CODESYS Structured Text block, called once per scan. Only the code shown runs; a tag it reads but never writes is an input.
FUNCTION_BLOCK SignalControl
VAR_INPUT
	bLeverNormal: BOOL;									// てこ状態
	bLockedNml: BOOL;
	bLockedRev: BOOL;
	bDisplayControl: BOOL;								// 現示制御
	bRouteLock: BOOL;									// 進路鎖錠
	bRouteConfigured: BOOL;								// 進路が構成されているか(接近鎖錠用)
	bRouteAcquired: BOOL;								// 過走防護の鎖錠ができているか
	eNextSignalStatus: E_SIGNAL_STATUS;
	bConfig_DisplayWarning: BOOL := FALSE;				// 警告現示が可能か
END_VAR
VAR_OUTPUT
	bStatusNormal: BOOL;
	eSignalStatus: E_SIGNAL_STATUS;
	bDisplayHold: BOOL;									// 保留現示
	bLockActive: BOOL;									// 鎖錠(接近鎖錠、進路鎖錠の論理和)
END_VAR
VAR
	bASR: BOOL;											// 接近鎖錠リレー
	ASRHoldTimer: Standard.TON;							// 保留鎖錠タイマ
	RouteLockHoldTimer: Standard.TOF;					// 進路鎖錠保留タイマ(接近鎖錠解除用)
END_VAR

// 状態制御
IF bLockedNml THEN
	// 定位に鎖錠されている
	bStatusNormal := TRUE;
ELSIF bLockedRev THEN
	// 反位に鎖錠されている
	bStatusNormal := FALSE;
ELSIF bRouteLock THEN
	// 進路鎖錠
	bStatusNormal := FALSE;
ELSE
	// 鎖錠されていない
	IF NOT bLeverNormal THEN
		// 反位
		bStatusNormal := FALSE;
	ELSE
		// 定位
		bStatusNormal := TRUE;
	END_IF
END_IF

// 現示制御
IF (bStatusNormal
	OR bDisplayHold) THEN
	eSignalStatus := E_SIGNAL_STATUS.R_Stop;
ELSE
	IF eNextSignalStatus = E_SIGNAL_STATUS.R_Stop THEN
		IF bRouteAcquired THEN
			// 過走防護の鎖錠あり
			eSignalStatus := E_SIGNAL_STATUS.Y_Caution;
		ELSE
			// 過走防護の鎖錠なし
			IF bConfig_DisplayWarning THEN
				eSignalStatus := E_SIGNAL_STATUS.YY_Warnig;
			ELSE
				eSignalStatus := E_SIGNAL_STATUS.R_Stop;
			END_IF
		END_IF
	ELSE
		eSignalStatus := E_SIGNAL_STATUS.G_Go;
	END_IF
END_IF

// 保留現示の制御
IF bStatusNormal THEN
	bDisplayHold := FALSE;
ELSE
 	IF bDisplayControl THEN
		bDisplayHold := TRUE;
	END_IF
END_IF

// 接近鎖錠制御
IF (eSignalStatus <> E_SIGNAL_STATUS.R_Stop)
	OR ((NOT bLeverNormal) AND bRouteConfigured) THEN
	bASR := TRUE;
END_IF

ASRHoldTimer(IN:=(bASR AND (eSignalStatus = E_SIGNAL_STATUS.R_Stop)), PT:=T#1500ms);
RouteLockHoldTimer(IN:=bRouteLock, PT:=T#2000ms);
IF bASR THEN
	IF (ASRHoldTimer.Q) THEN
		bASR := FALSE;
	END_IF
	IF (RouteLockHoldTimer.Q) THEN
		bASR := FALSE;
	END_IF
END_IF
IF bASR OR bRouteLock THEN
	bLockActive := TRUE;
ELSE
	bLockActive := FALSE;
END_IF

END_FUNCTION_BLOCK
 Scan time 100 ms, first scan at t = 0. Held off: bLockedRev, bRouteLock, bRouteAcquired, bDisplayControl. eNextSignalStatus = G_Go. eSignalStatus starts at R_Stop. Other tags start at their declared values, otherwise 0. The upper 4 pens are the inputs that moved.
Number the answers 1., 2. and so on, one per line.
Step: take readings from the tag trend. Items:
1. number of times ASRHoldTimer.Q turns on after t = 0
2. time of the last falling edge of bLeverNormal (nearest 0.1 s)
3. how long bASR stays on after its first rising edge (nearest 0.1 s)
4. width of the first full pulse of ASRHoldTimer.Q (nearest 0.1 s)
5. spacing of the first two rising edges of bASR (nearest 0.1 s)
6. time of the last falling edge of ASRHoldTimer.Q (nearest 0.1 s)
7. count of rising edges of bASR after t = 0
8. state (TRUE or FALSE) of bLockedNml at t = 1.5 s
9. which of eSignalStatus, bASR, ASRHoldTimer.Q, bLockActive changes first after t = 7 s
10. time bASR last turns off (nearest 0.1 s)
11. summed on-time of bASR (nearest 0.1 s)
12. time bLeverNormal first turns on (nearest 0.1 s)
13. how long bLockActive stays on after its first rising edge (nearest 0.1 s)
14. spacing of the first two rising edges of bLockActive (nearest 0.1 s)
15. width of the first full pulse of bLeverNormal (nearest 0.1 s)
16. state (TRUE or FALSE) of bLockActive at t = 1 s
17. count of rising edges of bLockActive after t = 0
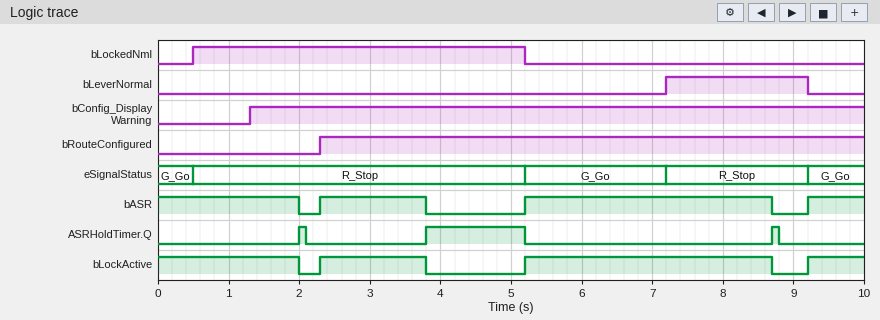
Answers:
1. 3
2. 9.2 s
3. 1.5 s
4. 0.1 s
5. 2.9 s
6. 8.8 s
7. 3
8. TRUE
9. eSignalStatus
10. 8.7 s
11. 7.8 s
12. 7.2 s
13. 1.5 s
14. 2.9 s
15. 2.0 s
16. TRUE
17. 3
